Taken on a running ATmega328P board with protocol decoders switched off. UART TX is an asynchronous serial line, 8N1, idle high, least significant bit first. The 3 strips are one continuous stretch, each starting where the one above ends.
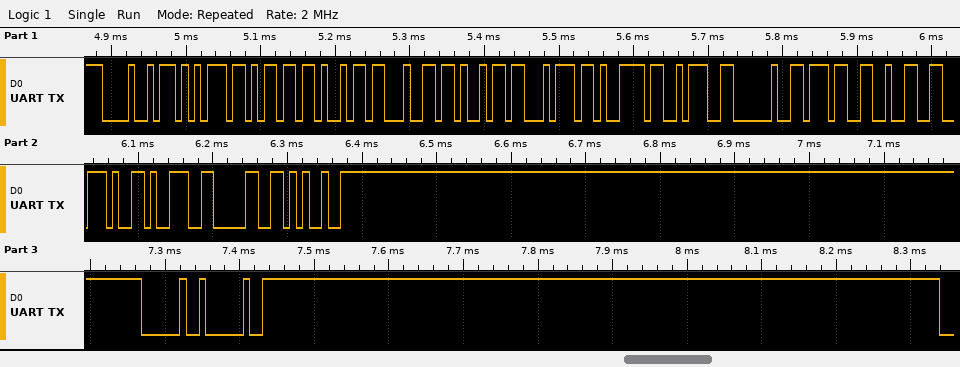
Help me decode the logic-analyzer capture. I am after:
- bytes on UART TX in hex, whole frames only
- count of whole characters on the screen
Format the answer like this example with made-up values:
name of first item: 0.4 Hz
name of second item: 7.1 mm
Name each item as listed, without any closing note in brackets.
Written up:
bytes on UART TX in hex, whole frames only: 48 75 6D 69 64 69 74 79 3A 20 37 32 2E 39 30 25 20 20
count of whole characters on the screen: 18
